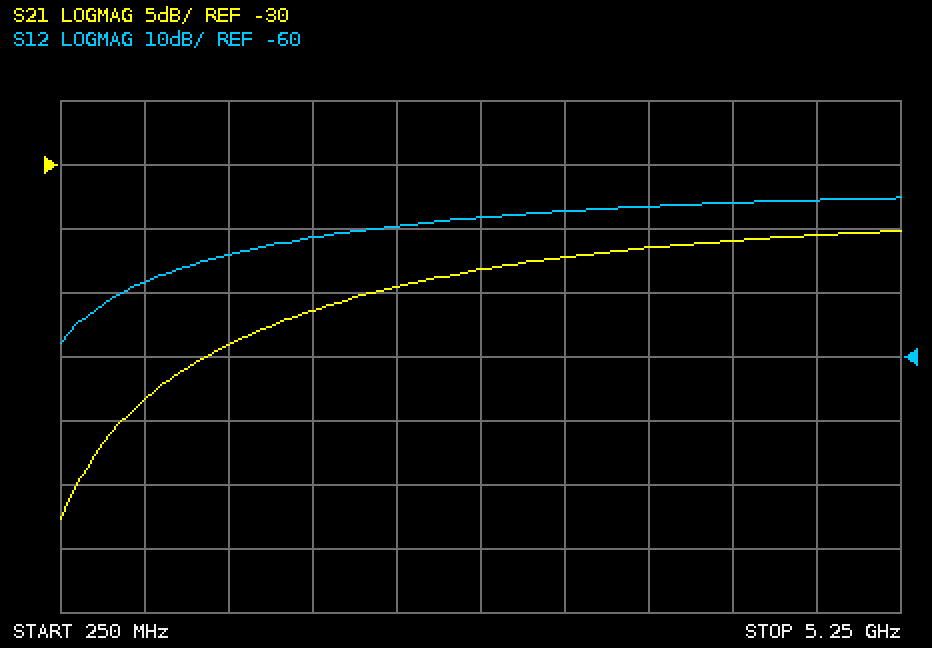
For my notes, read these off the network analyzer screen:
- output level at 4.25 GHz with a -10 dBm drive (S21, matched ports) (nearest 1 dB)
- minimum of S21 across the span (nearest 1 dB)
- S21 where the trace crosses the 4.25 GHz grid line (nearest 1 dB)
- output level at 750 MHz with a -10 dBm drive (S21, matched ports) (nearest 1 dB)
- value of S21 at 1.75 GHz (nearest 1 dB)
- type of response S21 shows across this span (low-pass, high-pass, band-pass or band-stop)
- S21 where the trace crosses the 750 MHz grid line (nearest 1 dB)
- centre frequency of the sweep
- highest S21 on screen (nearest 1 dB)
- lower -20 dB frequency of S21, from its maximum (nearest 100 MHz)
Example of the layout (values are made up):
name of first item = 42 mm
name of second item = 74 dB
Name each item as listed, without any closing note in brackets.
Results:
output level at 4.25 GHz with a -10 dBm drive (S21, matched ports) = -46 dBm
minimum of S21 across the span = -58 dB
S21 where the trace crosses the 4.25 GHz grid line = -36 dB
output level at 750 MHz with a -10 dBm drive (S21, matched ports) = -58 dBm
value of S21 at 1.75 GHz = -41 dB
type of response S21 shows across this span = high-pass
S21 where the trace crosses the 750 MHz grid line = -48 dB
centre frequency of the sweep = 2.75 GHz
highest S21 on screen = -35 dB
lower -20 dB frequency of S21, from its maximum = 300 MHz
